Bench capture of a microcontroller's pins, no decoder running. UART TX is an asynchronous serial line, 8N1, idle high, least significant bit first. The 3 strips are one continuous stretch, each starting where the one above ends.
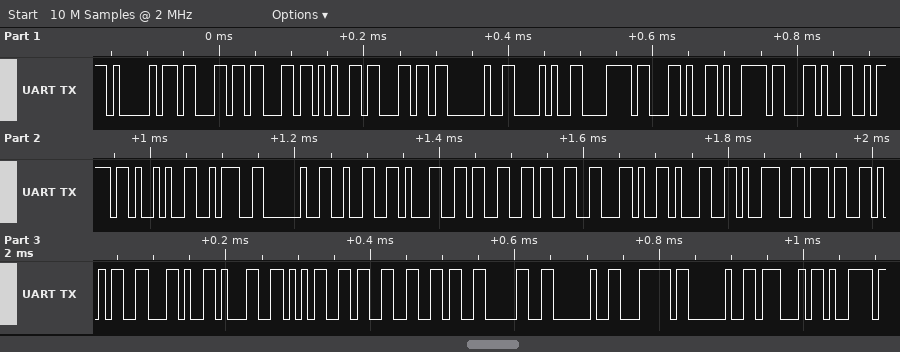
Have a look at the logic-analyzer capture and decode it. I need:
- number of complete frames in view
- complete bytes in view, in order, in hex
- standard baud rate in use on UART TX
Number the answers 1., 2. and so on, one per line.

1. 35
2. 41 63 63 65 6C 20 28 78 2C 79 2C 7A 29 3A 20 32 31 33 33 2C 31 39 37 35 2C 31 35 33 36 30 20 7C 20 47 79
3. 115200 baud
